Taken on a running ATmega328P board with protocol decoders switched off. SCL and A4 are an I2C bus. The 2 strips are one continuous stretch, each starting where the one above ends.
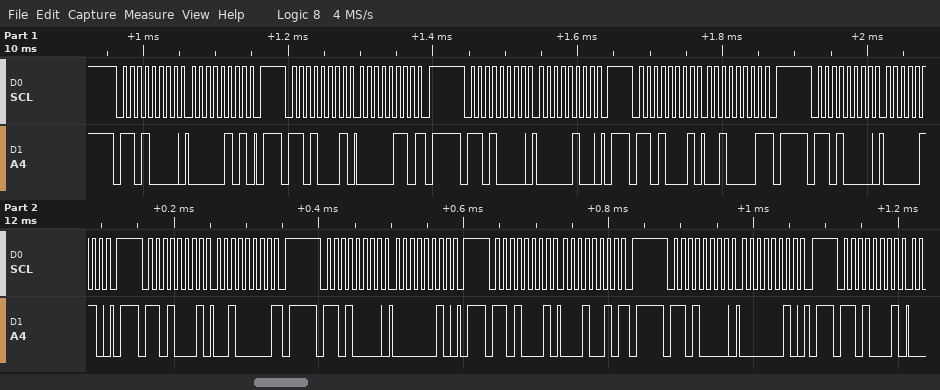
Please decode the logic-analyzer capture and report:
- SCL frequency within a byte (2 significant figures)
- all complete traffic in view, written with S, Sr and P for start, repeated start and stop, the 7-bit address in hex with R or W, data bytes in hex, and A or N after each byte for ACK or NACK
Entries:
100 kHz
S 68W A 05 A P S 68R A 06 N P S 68W A 04 A P S 68R A 21 N P S 68W A 06 A P S 68R A 20 N P S 68W A 02 A P S 68R A 12 N P S 68W A 02 A P S 68R A
